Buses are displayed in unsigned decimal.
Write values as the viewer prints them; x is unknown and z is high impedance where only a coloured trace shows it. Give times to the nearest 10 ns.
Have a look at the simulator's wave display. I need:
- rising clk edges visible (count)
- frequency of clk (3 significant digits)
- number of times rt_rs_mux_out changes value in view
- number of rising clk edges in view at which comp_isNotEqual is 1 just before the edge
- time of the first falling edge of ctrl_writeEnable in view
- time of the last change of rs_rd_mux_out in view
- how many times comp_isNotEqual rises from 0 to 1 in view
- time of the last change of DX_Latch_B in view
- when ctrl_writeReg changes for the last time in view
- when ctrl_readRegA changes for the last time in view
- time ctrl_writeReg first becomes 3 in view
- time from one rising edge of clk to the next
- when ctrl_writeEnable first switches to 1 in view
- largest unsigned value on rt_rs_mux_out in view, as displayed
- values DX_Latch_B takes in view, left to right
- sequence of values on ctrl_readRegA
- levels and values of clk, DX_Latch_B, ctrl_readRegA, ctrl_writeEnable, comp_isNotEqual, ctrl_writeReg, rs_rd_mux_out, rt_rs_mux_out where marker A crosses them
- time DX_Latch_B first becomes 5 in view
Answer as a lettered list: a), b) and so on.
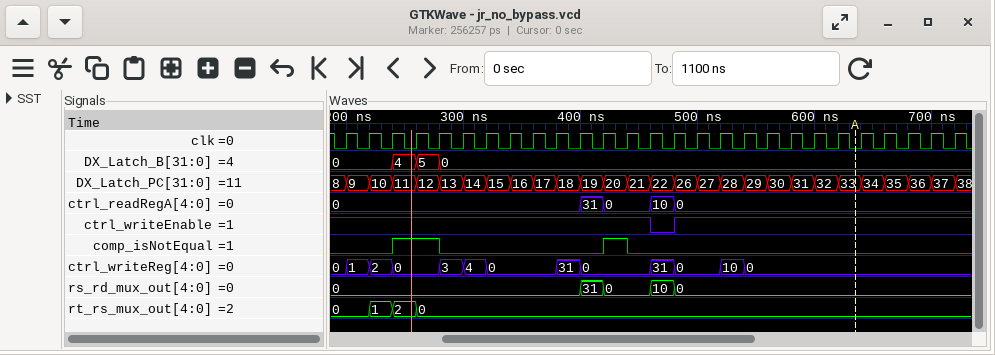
a) 27
b) 50.0 MHz
c) 3
d) 3
e) 460 ns
f) 480 ns
g) 2
h) 280 ns
i) 540 ns
j) 480 ns
k) 280 ns
l) 20 ns
m) 480 ns
n) 2
o) 0, 4, 5, 0
p) 0, 31, 0, 10, 0
q) clk=0, DX_Latch_B=0, ctrl_readRegA=0, ctrl_writeEnable=1, comp_isNotEqual=0, ctrl_writeReg=0, rs_rd_mux_out=0, rt_rs_mux_out=0
r) 260 ns
